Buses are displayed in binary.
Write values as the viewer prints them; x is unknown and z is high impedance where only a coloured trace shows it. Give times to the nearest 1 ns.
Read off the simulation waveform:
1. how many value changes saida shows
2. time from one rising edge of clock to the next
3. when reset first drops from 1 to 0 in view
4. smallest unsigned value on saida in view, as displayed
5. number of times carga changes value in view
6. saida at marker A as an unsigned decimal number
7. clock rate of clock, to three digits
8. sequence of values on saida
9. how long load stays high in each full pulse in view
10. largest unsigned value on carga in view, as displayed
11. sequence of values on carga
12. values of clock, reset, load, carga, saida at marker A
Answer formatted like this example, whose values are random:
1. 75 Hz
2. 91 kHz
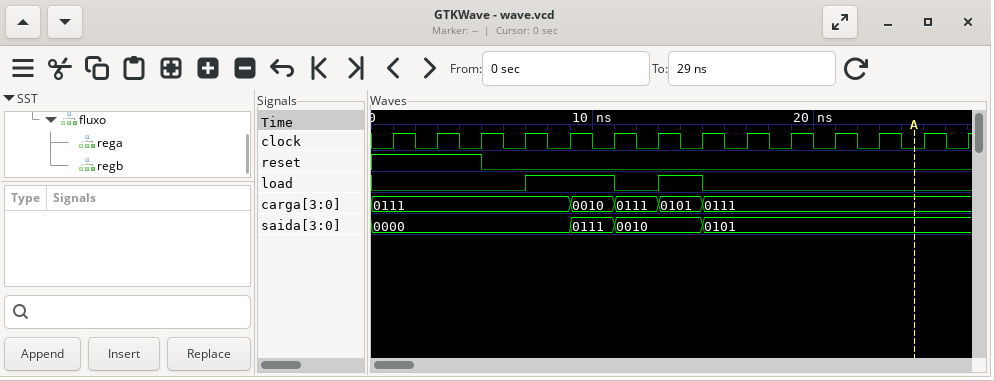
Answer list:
1. 3
2. 2 ns
3. 5 ns
4. 0000
5. 4
6. 5
7. 500 MHz
8. 0000, 0111, 0010, 0101
9. 4 ns, 2 ns
10. 0111
11. 0111, 0010, 0111, 0101, 0111
12. clock=0, reset=0, load=0, carga=0111, saida=0101
